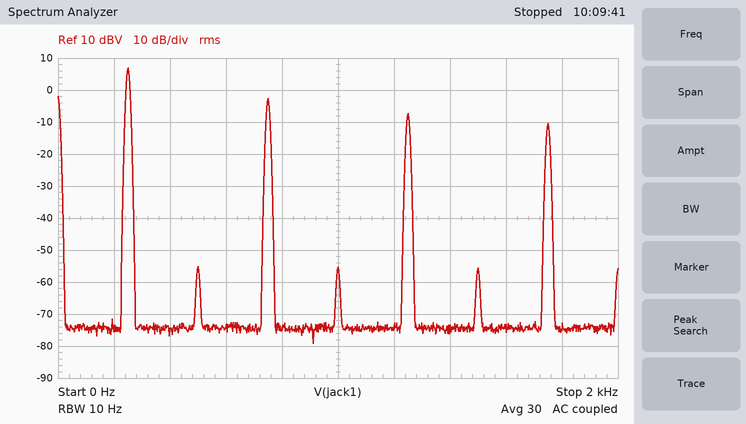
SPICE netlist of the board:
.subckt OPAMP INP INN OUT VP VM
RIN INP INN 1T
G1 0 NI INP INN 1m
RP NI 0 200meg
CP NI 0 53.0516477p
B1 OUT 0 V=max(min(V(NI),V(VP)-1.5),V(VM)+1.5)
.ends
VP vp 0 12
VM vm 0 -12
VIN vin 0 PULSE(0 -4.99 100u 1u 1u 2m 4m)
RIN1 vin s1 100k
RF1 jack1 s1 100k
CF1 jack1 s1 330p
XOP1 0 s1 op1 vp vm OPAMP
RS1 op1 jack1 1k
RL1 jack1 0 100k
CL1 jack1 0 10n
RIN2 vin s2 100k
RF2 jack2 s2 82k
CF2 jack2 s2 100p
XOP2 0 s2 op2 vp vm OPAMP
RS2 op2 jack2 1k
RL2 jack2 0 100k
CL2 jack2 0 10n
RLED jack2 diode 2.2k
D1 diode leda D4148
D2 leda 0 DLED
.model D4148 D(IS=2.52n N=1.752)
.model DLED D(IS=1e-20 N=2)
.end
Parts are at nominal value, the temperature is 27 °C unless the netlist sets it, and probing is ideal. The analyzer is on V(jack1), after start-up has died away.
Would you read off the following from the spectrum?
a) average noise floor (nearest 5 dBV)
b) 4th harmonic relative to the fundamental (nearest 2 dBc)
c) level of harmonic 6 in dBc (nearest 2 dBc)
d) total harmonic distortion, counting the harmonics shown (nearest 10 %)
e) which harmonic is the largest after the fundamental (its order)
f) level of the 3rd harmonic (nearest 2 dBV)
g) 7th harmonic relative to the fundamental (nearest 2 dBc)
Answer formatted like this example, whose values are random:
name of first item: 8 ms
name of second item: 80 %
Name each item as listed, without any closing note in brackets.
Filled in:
average noise floor: -75 dBV
4th harmonic relative to the fundamental: -62 dBc
level of harmonic 6 in dBc: -62 dBc
total harmonic distortion, counting the harmonics shown: 40 %
which harmonic is the largest after the fundamental: 3
level of the 3rd harmonic: -2 dBV
7th harmonic relative to the fundamental: -18 dBc
